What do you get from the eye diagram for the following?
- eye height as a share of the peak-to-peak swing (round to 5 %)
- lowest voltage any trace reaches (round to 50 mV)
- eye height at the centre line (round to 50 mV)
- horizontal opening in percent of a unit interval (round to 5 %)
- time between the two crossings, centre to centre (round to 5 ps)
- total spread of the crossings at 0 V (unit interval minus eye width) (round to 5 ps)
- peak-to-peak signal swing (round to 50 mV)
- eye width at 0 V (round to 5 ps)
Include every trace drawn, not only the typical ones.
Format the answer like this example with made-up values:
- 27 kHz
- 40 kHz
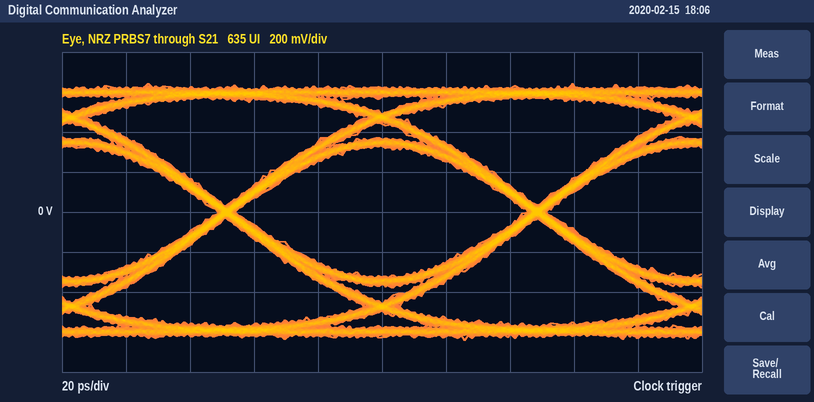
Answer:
- 50 %
- -650 mV
- 650 mV
- 95 %
- 95 ps
- 5 ps
- 1.30 V
- 90 ps
